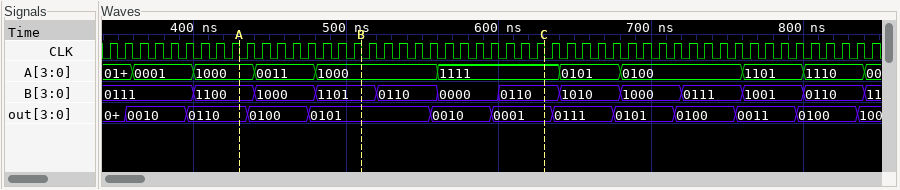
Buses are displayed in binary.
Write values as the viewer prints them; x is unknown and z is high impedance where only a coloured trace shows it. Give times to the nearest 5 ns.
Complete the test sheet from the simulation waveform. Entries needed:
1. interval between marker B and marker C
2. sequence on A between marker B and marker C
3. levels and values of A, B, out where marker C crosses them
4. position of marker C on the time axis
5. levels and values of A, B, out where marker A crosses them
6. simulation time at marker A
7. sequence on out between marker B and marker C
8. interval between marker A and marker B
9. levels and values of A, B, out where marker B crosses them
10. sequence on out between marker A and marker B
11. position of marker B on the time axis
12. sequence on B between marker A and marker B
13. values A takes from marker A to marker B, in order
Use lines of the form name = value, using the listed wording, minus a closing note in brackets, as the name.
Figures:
interval between marker B and marker C = 120 ns
sequence on A between marker B and marker C = 1000, 1111
levels and values of A, B, out where marker C crosses them = A=1111, B=0110, out=0001
position of marker C on the time axis = 630 ns
levels and values of A, B, out where marker A crosses them = A=1000, B=1100, out=0110
simulation time at marker A = 430 ns
sequence on out between marker B and marker C = 0101, 0010, 0001
interval between marker A and marker B = 80 ns
levels and values of A, B, out where marker B crosses them = A=1000, B=1101, out=0101
sequence on out between marker A and marker B = 0110, 0100, 0101
position of marker B on the time axis = 510 ns
sequence on B between marker A and marker B = 1100, 1000, 1101
values A takes from marker A to marker B, in order = 1000, 0011, 1000
